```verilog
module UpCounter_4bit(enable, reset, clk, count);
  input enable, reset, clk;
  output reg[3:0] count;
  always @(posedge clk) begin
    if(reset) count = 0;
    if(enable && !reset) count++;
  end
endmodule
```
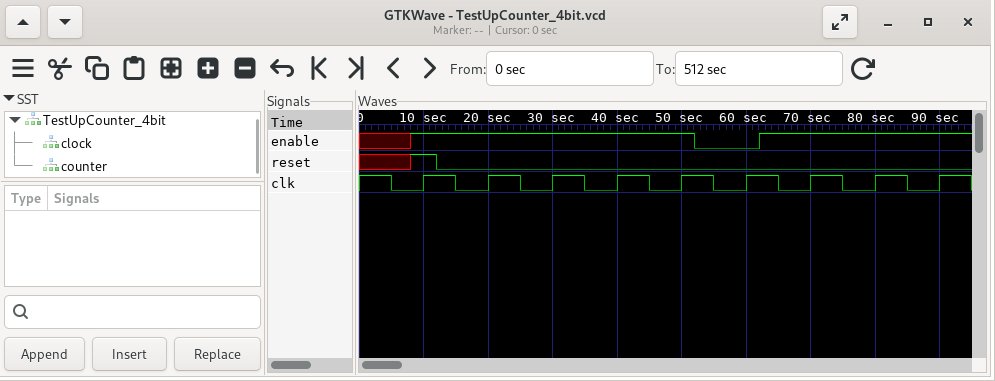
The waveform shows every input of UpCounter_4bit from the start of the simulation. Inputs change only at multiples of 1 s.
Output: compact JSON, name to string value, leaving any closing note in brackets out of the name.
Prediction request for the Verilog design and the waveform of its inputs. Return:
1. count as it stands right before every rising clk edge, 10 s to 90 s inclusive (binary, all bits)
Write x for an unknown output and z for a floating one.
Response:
{"count as it stands right before every rising clk edge, 10 s to 90 s inclusive": "x, 0000, 0001, 0010, 0011, 0100, 0100, 0101, 0110"}
